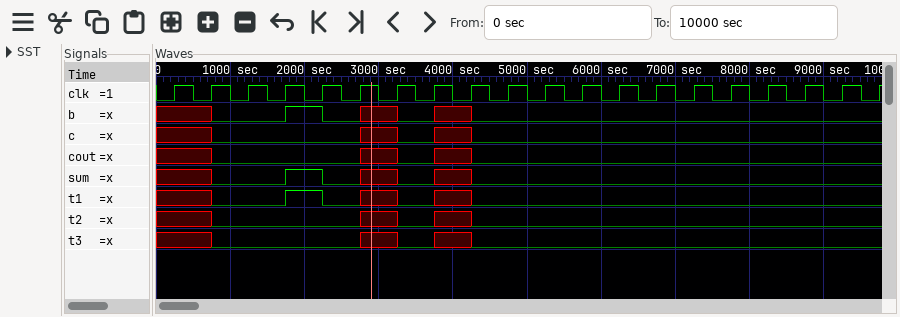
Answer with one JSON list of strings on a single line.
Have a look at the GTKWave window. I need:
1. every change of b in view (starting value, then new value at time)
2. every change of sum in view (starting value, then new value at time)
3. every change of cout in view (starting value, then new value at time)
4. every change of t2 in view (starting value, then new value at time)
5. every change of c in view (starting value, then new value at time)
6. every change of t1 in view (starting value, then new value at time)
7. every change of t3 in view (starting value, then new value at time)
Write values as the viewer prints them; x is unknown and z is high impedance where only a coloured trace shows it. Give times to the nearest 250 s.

["x, 0 at 750 s, 1 at 1750 s, 0 at 2250 s, x at 2750 s, 0 at 3250 s, x at 3750 s, 0 at 4250 s", "x, 0 at 750 s, 1 at 1750 s, 0 at 2250 s, x at 2750 s, 0 at 3250 s, x at 3750 s, 0 at 4250 s", "x, 0 at 750 s, x at 2750 s, 0 at 3250 s, x at 3750 s, 0 at 4250 s", "x, 0 at 750 s, x at 2750 s, 0 at 3250 s, x at 3750 s, 0 at 4250 s", "x, 0 at 750 s, x at 2750 s, 0 at 3250 s, x at 3750 s, 0 at 4250 s", "x, 0 at 750 s, 1 at 1750 s, 0 at 2250 s, x at 2750 s, 0 at 3250 s, x at 3750 s, 0 at 4250 s", "x, 0 at 750 s, x at 2750 s, 0 at 3250 s, x at 3750 s, 0 at 4250 s"]
